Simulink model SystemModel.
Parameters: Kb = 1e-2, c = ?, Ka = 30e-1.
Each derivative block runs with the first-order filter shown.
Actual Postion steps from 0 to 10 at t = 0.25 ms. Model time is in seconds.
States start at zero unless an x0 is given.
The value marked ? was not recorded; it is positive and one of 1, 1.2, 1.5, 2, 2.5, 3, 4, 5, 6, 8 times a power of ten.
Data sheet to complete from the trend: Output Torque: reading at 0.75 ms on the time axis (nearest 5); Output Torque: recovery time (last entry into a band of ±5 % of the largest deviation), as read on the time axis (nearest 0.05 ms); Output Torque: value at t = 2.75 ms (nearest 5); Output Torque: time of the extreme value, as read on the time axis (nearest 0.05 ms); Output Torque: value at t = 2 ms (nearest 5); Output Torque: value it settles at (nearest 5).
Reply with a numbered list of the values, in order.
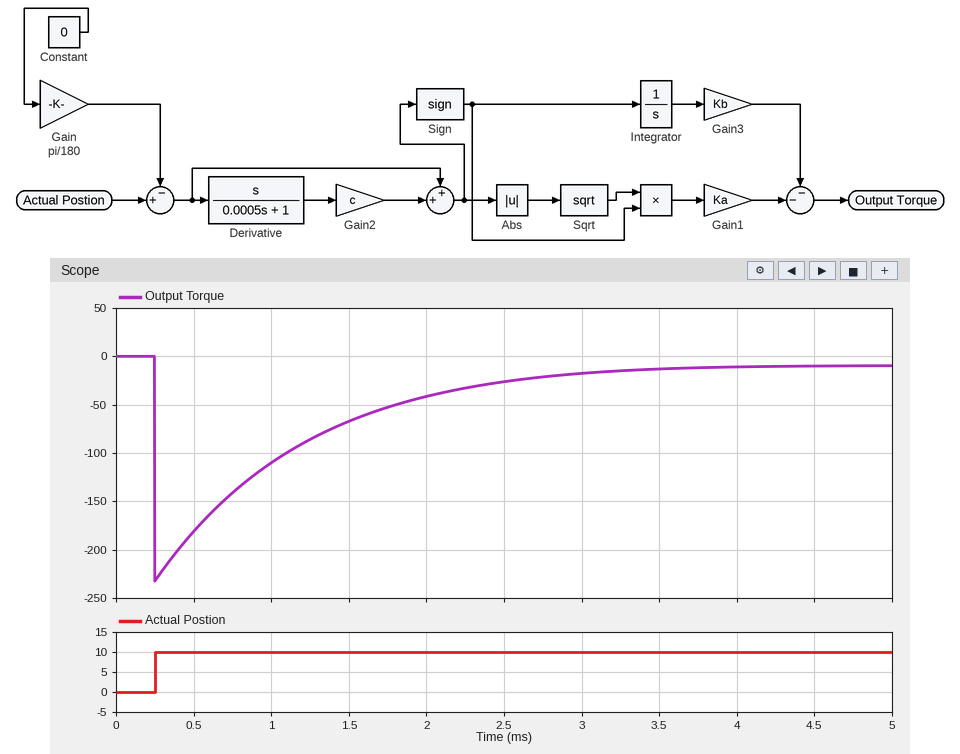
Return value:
1. -140
2. 2.75 ms
3. -20
4. 0.25 ms
5. -40
6. -10
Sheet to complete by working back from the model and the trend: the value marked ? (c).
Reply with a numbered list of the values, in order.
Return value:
1. 0.3
